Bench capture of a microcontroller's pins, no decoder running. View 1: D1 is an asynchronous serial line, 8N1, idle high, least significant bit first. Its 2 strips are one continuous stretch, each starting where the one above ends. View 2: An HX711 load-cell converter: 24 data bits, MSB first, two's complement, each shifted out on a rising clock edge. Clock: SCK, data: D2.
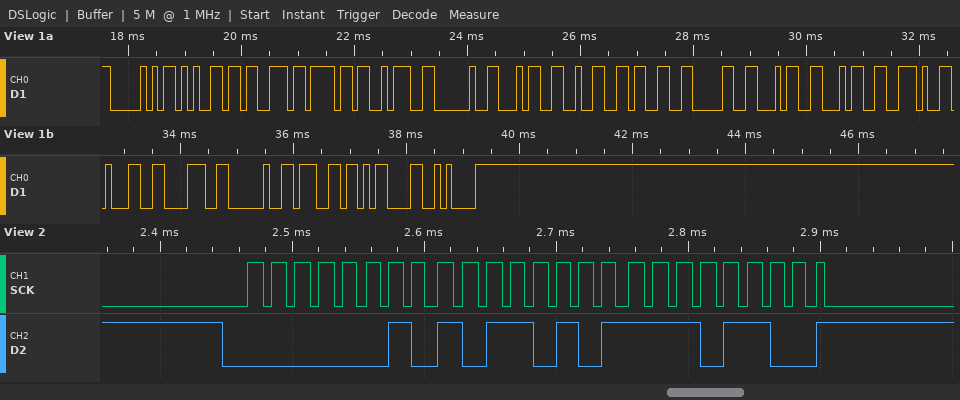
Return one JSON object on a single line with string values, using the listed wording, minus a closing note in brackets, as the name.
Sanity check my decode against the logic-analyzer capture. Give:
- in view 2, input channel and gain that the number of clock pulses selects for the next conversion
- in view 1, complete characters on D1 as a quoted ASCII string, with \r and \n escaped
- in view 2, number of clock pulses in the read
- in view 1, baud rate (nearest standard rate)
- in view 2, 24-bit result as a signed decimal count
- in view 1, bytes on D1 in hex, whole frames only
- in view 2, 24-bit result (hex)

{"in view 2, input channel and gain that the number of clock pulses selects for the next conversion": "channel A, gain 128", "in view 1, complete characters on D1 as a quoted ASCII string, with \\r and \\n escaped": "\"Peso: 423044.18 g\\r\\n\"", "in view 2, number of clock pulses in the read": "25", "in view 1, baud rate": "9600 baud", "in view 2, 24-bit result as a signed decimal count": "177644", "in view 1, bytes on D1 in hex, whole frames only": "0x50 0x65 0x73 0x6F 0x3A 0x20 0x34 0x32 0x33 0x30 0x34 0x34 0x2E 0x31 0x38 0x20 0x67 0x0D 0x0A", "in view 2, 24-bit result": "0x02B5EC"}
